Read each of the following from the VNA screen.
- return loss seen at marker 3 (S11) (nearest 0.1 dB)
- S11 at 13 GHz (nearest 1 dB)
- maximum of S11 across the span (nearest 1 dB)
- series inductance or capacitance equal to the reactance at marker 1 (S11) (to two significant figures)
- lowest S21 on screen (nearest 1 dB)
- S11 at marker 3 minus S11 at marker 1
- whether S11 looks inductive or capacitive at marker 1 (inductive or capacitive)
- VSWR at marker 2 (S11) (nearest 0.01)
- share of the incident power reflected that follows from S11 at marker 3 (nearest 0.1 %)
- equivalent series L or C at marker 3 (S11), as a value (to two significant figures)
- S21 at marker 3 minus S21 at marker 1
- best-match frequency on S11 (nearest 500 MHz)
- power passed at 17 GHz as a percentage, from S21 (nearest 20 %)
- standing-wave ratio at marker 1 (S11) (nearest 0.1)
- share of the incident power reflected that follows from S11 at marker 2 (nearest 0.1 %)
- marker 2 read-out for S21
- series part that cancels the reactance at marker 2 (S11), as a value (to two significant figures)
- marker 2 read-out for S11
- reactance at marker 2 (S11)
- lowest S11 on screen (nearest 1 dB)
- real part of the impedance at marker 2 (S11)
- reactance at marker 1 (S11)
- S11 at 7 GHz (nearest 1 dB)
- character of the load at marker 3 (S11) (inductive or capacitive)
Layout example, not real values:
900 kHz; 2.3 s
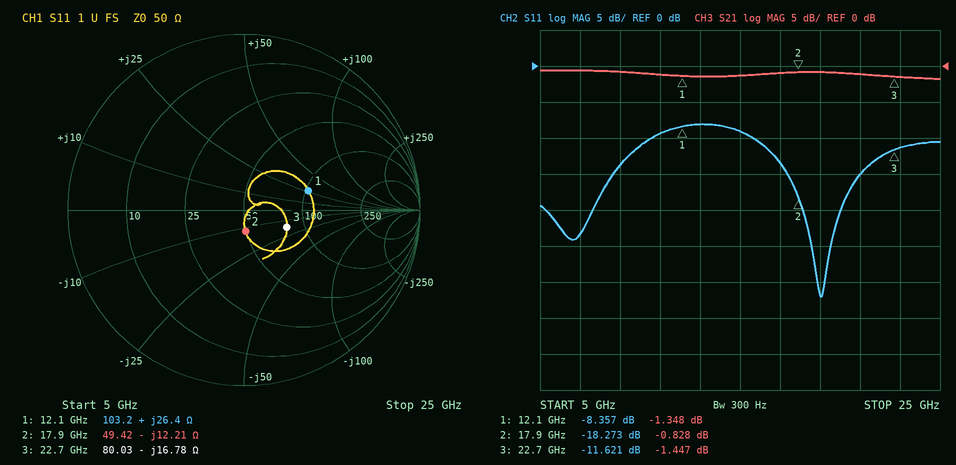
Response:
11.6 dB; -8 dB; -8 dB; 350 pH; -2 dB; -3.264 dB; inductive; 1.28; 6.9 %; 420 fF; -0.099 dB; 19.0 GHz; 80 %; 2.2; 1.5 %; -0.828 dB; 110 pH; -18.273 dB; -12.21 Ω; -32 dB; 49.42 Ω; +26.4 Ω; -23 dB; capacitive
